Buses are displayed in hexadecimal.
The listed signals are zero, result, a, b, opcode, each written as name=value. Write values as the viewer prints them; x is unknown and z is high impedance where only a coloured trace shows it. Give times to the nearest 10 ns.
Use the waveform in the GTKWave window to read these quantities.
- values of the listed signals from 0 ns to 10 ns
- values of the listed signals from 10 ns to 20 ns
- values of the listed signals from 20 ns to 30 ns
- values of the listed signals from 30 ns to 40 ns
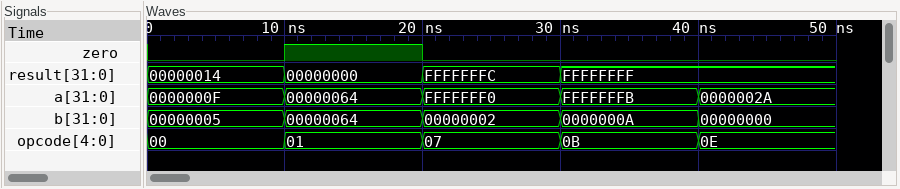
zero=0, result=00000014, a=0000000F, b=00000005, opcode=00
zero=1, result=00000000, a=00000064, b=00000064, opcode=01
zero=0, result=FFFFFFFC, a=FFFFFFF0, b=00000002, opcode=07
zero=0, result=FFFFFFFF, a=FFFFFFFB, b=0000000A, opcode=0B
